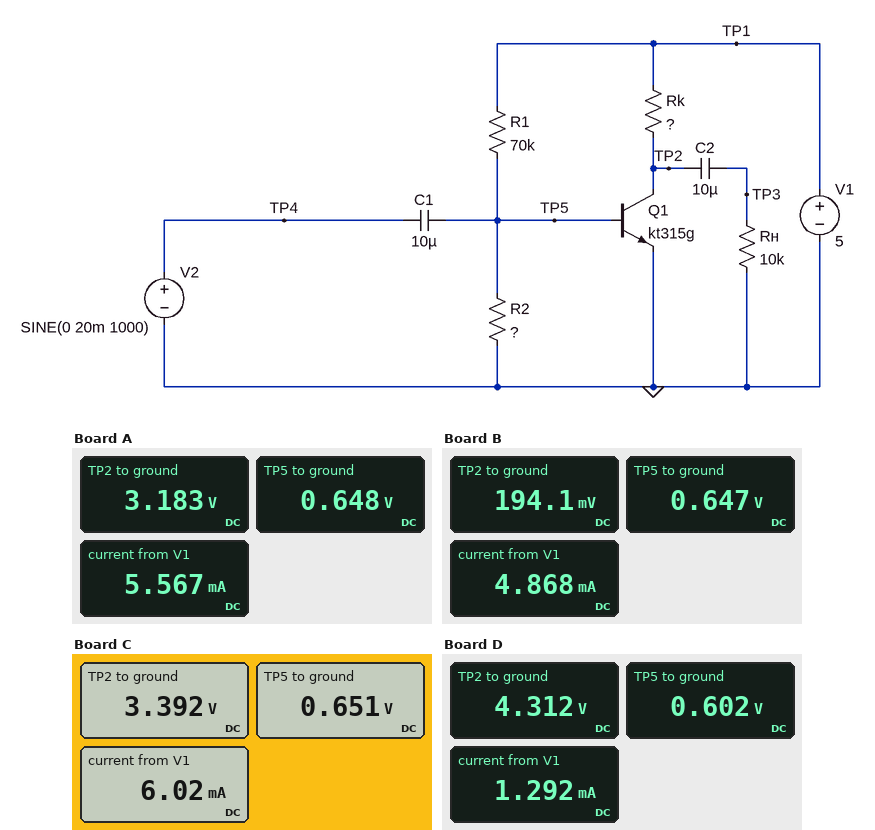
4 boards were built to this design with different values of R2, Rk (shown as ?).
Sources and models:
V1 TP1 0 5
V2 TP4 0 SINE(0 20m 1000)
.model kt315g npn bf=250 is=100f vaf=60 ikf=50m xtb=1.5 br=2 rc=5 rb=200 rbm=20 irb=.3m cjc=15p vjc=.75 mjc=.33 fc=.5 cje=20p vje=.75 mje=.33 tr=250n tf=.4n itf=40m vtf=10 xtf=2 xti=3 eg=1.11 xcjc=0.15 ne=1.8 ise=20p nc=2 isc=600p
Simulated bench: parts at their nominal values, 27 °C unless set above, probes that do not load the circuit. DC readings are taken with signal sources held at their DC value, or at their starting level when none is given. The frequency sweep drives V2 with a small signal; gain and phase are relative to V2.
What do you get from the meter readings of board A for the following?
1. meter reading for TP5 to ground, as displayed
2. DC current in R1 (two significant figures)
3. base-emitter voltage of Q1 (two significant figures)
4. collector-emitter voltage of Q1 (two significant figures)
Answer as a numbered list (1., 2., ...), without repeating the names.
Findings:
1. 0.648 V
2. 62 µA
3. 650 mV
4. 3.2 V
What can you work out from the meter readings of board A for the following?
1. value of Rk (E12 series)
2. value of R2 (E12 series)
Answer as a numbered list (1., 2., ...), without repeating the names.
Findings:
1. 330 Ω
2. 33 kΩ
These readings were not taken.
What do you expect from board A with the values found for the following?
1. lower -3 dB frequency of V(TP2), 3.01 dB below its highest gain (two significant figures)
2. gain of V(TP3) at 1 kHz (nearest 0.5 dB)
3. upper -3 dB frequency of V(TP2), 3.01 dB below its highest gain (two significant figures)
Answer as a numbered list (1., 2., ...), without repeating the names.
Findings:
1. 18 Hz
2. 34.0 dB
3. 5.6 MHz
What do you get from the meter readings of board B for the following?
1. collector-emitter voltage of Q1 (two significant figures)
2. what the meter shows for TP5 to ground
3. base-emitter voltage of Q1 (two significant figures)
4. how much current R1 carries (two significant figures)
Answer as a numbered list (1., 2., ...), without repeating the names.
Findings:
1. 190 mV
2. 0.647 V
3. 650 mV
4. 62 µA
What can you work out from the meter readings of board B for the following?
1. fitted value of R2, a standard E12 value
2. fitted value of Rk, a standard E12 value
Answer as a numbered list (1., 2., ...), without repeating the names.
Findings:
1. 47 kΩ
2. 1 kΩ
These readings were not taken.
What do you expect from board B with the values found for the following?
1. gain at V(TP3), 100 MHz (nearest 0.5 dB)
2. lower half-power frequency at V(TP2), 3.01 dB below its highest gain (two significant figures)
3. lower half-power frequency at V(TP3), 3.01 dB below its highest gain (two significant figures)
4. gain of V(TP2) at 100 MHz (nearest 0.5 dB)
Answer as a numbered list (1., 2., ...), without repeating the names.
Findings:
1. -12.5 dB
2. 80 Hz
3. 80 Hz
4. -12.5 dB
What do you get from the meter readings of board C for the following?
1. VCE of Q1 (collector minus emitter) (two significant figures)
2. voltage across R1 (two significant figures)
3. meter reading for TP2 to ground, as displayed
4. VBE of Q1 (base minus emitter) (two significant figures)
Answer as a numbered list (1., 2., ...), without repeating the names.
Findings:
1. 3.4 V
2. 4.3 V
3. 3.392 V
4. 650 mV
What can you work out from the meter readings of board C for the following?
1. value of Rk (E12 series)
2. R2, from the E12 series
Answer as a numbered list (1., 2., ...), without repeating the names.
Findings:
1. 270 Ω
2. 39 kΩ
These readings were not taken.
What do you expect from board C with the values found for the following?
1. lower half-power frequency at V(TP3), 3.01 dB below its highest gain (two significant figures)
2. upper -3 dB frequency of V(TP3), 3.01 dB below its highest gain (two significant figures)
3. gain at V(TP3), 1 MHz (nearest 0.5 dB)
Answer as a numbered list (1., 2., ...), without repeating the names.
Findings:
1. 19 Hz
2. 5.9 MHz
3. 32.5 dB
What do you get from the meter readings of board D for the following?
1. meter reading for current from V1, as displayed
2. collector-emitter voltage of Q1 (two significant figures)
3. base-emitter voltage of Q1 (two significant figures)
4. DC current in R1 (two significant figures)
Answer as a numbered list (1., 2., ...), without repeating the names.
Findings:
1. 1.292 mA
2. 4.3 V
3. 600 mV
4. 63 µA
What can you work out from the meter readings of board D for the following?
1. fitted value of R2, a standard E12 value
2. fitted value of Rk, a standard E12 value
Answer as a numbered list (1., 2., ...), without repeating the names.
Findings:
1. 12 kΩ
2. 560 Ω
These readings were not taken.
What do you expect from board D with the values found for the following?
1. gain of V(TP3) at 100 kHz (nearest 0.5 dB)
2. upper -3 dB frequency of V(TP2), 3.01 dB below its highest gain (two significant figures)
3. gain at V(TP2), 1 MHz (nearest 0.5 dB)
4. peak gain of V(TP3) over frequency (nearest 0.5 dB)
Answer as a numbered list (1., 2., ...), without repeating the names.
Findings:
1. 27.0 dB
2. 9.8 MHz
3. 27.0 dB
4. 27.0 dB
